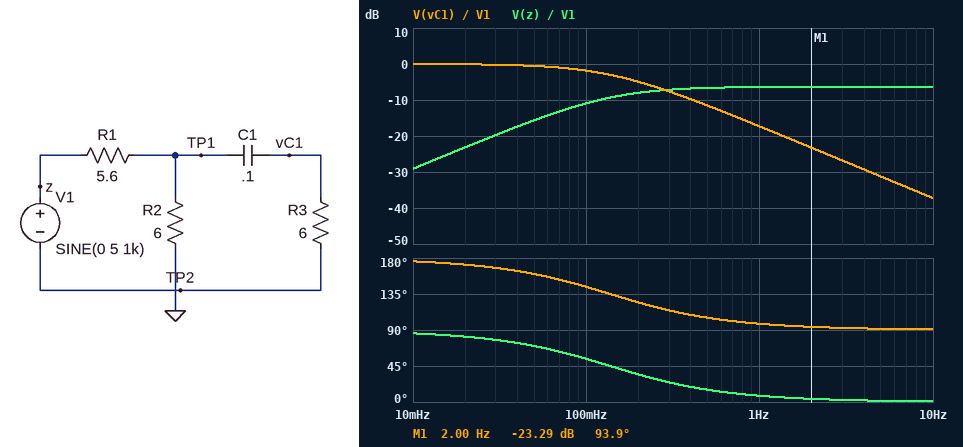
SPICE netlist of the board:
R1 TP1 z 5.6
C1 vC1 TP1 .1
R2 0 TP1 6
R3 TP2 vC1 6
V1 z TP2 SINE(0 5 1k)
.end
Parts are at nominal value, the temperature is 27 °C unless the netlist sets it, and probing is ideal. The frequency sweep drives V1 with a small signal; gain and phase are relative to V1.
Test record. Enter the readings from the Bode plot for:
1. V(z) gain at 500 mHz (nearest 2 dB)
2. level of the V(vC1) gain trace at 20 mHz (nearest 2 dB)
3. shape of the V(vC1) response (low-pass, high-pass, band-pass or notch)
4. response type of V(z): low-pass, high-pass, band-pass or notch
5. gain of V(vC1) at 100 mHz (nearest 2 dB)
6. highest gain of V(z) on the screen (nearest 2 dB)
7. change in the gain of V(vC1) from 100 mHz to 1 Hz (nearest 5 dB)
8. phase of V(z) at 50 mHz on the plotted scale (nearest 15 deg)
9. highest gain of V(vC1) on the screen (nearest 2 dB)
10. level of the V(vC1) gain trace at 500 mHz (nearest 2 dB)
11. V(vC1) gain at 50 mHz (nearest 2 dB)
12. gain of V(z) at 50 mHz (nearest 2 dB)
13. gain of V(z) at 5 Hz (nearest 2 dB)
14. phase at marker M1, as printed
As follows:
-6 dB
0 dB
low-pass
high-pass
-2 dB
-6 dB
-15 dB
75 deg
0 dB
-12 dB
0 dB
-16 dB
-6 dB
93.9 deg
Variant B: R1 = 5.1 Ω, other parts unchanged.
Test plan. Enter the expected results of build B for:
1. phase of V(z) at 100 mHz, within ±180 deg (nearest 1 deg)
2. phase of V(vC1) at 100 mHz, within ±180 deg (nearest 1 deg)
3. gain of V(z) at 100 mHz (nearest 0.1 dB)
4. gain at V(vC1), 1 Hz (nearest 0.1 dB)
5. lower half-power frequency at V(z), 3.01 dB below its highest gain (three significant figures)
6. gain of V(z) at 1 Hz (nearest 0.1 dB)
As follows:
55 deg
145 deg
-11.6 dB
-17.0 dB
143 mHz
-6.8 dB
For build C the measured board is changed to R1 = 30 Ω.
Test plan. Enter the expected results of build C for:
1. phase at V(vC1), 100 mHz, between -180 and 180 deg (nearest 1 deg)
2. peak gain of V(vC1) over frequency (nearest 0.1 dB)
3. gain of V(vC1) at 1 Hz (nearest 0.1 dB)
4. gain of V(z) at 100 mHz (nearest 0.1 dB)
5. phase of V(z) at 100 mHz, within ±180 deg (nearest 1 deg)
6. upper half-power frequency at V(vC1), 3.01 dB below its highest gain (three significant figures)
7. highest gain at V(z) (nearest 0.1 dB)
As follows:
114 deg
0 dB
-27.1 dB
-2.4 dB
24 deg
44.2 mHz
-1.6 dB
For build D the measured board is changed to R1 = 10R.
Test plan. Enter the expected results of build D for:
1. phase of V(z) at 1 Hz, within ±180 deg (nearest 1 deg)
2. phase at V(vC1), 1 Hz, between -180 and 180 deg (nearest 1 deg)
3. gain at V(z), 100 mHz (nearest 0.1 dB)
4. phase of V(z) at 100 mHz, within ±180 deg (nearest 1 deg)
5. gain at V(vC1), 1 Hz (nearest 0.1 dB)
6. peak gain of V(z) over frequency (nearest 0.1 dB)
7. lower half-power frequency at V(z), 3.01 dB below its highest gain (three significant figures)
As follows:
6 deg
96 deg
-7.1 dB
45 deg
-20.1 dB
-4.1 dB
99.5 mHz
